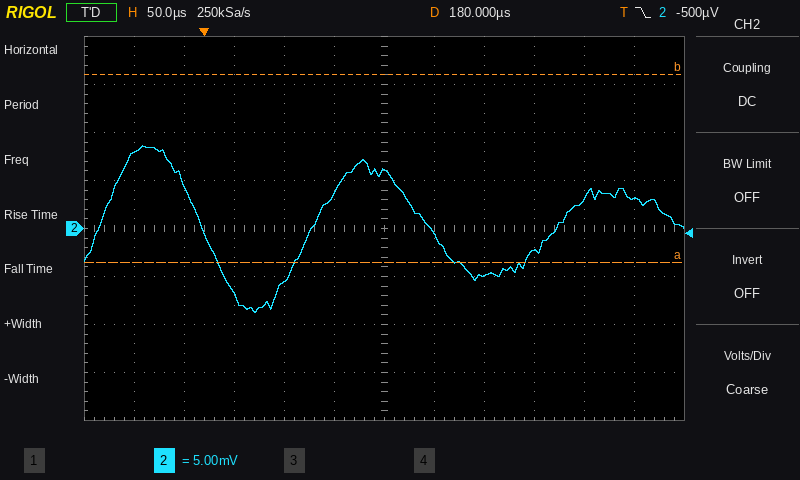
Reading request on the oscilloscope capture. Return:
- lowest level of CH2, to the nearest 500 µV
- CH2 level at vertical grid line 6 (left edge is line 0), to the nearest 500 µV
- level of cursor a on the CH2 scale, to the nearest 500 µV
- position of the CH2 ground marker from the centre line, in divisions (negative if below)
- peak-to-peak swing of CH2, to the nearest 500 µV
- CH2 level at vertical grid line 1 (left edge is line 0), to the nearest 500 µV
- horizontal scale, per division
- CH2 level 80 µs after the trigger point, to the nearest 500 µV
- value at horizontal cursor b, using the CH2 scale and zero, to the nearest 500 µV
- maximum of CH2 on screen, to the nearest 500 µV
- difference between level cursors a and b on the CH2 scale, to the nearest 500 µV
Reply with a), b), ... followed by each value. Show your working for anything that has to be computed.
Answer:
a) -9.0 mV
b) 6.0 mV
c) -3.5 mV
d) 0.0 div
e) 8.5 mV − (-9.0 mV) = 17.5 mV
f) 8.0 mV
g) 50 µs
h) -5.5 mV
i) 16.0 mV
j) 8.5 mV
k) 19.5 mV
